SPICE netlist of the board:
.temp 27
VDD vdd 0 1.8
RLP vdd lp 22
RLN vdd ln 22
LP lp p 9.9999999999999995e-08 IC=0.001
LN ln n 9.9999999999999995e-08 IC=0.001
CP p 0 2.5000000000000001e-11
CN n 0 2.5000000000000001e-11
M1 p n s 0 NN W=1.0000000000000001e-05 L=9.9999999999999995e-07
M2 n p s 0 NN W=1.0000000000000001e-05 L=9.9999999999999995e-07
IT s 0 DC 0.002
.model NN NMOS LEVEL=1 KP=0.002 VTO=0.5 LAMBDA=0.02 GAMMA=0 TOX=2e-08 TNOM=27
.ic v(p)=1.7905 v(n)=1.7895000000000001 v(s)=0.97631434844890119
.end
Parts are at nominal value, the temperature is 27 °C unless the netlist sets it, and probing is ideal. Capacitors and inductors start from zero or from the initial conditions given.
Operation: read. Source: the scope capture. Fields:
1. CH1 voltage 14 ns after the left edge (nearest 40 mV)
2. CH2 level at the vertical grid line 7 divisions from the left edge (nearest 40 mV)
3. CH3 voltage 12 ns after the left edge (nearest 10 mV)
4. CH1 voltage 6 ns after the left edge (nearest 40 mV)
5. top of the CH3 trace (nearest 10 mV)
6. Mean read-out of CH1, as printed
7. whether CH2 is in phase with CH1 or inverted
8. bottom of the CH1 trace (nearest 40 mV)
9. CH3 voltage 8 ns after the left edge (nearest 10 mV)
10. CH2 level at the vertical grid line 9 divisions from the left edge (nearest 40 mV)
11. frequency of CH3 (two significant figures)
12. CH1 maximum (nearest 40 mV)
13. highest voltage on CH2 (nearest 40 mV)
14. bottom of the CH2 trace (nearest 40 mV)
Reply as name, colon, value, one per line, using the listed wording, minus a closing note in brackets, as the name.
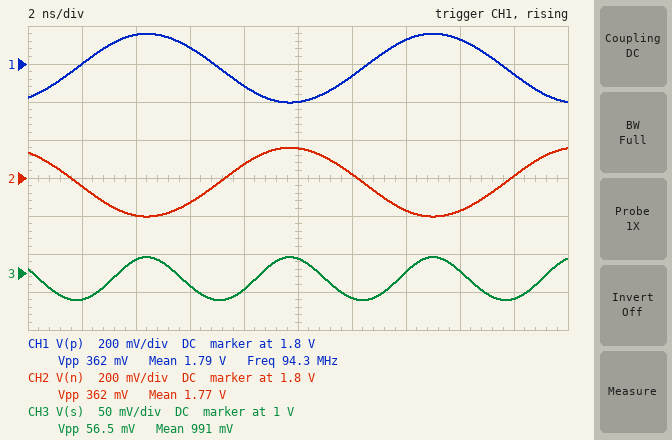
CH1 voltage 14 ns after the left edge: 1.92 V
CH2 level at the vertical grid line 7 divisions from the left edge: 1.64 V
CH3 voltage 12 ns after the left edge: 970 mV
CH1 voltage 6 ns after the left edge: 1.88 V
top of the CH3 trace: 1.02 V
Mean read-out of CH1, as printed: 1.79 V
whether CH2 is in phase with CH1 or inverted: inverted
bottom of the CH1 trace: 1.60 V
CH3 voltage 8 ns after the left edge: 980 mV
CH2 level at the vertical grid line 9 divisions from the left edge: 1.80 V
frequency of CH3: 190 MHz
CH1 maximum: 1.96 V
highest voltage on CH2: 1.96 V
bottom of the CH2 trace: 1.60 V
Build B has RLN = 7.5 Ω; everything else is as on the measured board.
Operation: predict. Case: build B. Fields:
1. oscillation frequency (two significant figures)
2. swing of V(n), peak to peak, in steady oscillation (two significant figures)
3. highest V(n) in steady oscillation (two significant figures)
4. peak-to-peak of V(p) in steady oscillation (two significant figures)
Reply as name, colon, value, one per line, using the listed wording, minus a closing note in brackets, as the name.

oscillation frequency: 99 MHz
swing of V(n), peak to peak, in steady oscillation: 1.3 V
highest V(n) in steady oscillation: 2.4 V
peak-to-peak of V(p) in steady oscillation: 470 mV
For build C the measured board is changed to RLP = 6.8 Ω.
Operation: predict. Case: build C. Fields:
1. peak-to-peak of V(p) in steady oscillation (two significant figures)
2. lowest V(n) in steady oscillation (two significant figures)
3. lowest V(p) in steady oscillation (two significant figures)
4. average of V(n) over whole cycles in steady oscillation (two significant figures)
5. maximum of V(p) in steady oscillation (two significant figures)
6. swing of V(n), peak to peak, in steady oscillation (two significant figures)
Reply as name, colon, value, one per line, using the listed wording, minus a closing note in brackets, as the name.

peak-to-peak of V(p) in steady oscillation: 1.4 V
lowest V(n) in steady oscillation: 1.5 V
lowest V(p) in steady oscillation: 1.1 V
average of V(n) over whole cycles in steady oscillation: 1.8 V
maximum of V(p) in steady oscillation: 2.5 V
swing of V(n), peak to peak, in steady oscillation: 470 mV
